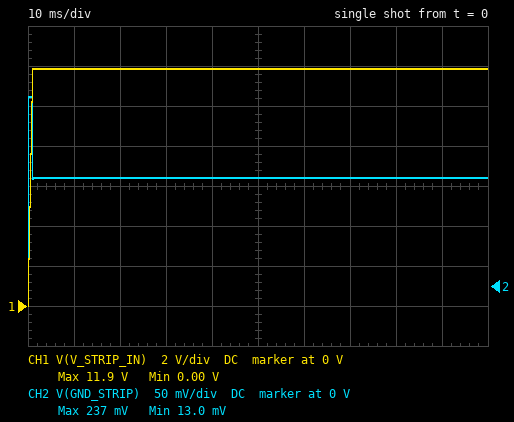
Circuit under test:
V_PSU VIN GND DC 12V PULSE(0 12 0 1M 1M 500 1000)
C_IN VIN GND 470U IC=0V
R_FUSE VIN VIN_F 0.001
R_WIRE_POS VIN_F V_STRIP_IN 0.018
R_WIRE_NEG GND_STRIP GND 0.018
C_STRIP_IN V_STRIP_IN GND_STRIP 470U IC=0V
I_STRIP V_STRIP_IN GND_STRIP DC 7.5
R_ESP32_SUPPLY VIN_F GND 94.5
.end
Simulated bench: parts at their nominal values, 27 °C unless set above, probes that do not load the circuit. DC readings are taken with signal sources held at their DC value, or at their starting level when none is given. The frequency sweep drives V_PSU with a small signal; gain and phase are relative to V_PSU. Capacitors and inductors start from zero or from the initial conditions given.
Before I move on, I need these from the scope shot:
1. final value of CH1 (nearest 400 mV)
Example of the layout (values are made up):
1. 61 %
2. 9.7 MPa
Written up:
1. 12.0 V
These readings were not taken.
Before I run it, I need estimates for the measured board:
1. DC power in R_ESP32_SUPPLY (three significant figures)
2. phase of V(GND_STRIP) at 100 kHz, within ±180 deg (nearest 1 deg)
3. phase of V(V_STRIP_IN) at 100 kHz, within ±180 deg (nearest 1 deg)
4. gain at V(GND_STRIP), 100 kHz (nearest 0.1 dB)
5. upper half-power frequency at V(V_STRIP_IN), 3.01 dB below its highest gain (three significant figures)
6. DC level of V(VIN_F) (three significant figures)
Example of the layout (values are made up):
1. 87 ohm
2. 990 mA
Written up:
1. 1.52 W
2. 5 deg
3. -5 deg
4. -6.3 dB
5. 12.6 kHz
6. 12.0 V
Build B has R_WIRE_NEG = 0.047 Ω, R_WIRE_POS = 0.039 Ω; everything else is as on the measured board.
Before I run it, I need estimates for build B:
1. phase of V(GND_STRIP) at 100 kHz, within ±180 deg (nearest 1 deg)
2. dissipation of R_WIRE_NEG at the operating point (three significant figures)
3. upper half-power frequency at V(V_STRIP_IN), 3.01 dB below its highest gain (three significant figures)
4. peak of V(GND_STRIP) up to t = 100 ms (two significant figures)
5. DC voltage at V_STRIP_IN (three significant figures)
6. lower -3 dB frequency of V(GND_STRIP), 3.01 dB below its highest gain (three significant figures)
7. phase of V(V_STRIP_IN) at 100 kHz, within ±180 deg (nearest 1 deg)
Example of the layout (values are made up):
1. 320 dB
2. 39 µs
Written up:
1. 2 deg
2. 2.64 W
3. 6.03 kHz
4. 620 mV
5. 11.7 V
6. 3.89 kHz
7. -2 deg
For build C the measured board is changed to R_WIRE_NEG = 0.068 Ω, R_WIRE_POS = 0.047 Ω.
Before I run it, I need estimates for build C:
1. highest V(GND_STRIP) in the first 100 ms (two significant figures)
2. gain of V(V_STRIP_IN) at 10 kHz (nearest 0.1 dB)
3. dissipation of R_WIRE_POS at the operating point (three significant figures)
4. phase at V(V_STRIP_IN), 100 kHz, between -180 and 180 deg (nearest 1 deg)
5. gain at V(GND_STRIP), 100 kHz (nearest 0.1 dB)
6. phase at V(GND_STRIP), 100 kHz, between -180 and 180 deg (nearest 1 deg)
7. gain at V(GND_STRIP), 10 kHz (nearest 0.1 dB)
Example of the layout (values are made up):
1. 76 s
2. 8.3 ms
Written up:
1. 890 mV
2. -4.0 dB
3. 2.64 W
4. -1 deg
5. -4.6 dB
6. 2 deg
7. -5.0 dB
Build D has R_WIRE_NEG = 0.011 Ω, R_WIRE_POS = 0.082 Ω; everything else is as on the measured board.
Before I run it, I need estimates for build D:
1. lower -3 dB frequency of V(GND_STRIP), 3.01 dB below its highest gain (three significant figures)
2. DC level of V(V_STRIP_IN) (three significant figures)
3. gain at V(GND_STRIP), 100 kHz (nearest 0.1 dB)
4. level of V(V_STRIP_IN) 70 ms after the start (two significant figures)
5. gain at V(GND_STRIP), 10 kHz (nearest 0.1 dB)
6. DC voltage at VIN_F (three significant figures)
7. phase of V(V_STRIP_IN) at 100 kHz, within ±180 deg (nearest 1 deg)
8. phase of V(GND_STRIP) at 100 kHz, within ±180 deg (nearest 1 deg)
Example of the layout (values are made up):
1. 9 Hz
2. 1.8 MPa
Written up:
1. 3.60 kHz
2. 11.4 V
3. -18.6 dB
4. 11 V
5. -19.2 dB
6. 12.0 V
7. -15 deg
8. 2 deg
